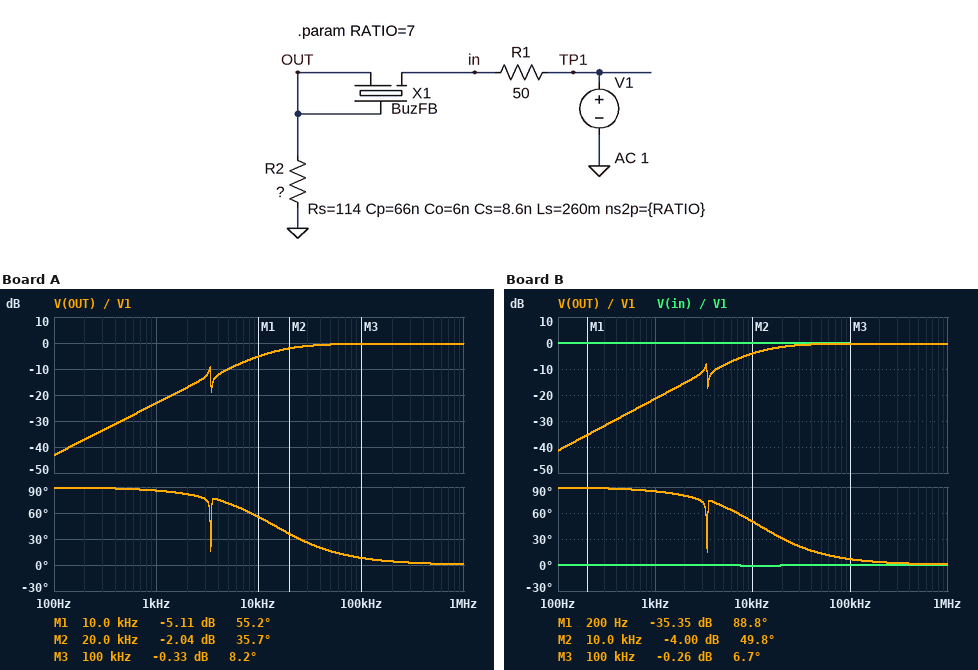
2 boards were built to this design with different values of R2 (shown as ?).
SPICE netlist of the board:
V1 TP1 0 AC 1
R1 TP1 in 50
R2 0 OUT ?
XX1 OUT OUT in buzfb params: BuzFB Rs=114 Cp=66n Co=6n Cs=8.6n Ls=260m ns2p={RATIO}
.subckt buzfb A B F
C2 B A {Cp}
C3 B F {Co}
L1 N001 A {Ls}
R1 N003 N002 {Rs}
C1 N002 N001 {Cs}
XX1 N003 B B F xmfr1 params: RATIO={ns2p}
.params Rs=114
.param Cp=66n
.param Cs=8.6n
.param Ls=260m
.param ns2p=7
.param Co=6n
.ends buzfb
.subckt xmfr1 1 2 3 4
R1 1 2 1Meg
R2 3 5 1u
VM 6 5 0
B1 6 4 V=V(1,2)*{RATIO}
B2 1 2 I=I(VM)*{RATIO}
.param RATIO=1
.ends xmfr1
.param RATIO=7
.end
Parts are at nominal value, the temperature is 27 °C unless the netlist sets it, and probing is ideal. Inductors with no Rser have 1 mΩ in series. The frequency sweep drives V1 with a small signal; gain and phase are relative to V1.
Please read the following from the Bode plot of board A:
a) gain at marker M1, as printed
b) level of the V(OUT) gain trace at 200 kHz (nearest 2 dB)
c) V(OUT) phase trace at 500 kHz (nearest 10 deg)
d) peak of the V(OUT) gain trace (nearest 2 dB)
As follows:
-5.11 dB
0 dB
0 deg
0 dB
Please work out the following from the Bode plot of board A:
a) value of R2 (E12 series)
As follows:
1.8 kΩ
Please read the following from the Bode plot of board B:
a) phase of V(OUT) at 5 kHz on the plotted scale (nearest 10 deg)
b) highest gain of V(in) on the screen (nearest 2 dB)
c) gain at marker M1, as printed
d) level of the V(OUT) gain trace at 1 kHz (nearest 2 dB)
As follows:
70 deg
0 dB
-35.35 dB
-22 dB
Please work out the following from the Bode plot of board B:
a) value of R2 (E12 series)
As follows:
2.2 kΩ
